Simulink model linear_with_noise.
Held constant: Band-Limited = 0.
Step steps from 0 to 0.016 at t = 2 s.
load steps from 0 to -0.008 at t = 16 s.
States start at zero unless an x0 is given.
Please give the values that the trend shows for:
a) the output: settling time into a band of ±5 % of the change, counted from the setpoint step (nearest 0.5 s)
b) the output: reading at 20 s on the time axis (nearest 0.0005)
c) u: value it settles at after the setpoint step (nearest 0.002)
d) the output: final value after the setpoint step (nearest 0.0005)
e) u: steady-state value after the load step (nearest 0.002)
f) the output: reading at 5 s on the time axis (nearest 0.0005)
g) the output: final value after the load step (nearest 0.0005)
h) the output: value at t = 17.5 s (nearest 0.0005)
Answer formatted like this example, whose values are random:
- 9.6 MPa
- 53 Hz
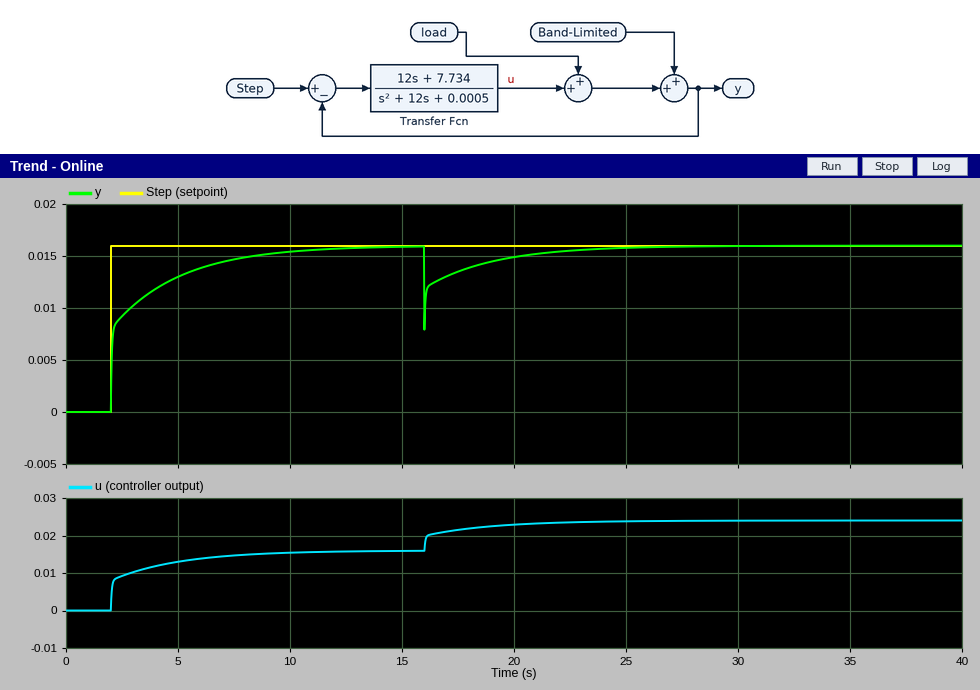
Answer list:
- 7.0 s
- 0.0150
- 0.016
- 0.0160
- 0.024
- 0.0130
- 0.0160
- 0.0135
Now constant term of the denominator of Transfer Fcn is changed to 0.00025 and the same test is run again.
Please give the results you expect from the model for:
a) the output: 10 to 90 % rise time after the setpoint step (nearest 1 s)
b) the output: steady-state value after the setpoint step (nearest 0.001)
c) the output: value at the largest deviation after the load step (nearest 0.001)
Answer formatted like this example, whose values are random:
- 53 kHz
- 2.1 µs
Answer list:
- 5 s
- 0.016
- 0.008
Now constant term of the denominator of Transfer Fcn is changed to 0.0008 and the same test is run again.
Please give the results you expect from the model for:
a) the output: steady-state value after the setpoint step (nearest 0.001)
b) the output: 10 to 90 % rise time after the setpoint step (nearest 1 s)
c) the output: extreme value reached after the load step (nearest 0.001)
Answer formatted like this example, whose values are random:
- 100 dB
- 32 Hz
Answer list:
- 0.016
- 5 s
- 0.008
